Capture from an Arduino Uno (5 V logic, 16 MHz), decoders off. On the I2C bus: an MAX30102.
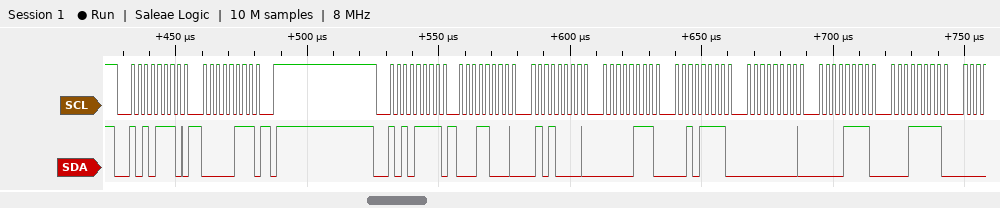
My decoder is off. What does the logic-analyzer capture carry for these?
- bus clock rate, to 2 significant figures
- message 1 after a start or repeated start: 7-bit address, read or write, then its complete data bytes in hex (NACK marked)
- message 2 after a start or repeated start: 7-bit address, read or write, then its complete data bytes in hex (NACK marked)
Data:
400 kHz
0x57 write: 07
0x57 read: 18 50 07 2F 00 0F 1F
